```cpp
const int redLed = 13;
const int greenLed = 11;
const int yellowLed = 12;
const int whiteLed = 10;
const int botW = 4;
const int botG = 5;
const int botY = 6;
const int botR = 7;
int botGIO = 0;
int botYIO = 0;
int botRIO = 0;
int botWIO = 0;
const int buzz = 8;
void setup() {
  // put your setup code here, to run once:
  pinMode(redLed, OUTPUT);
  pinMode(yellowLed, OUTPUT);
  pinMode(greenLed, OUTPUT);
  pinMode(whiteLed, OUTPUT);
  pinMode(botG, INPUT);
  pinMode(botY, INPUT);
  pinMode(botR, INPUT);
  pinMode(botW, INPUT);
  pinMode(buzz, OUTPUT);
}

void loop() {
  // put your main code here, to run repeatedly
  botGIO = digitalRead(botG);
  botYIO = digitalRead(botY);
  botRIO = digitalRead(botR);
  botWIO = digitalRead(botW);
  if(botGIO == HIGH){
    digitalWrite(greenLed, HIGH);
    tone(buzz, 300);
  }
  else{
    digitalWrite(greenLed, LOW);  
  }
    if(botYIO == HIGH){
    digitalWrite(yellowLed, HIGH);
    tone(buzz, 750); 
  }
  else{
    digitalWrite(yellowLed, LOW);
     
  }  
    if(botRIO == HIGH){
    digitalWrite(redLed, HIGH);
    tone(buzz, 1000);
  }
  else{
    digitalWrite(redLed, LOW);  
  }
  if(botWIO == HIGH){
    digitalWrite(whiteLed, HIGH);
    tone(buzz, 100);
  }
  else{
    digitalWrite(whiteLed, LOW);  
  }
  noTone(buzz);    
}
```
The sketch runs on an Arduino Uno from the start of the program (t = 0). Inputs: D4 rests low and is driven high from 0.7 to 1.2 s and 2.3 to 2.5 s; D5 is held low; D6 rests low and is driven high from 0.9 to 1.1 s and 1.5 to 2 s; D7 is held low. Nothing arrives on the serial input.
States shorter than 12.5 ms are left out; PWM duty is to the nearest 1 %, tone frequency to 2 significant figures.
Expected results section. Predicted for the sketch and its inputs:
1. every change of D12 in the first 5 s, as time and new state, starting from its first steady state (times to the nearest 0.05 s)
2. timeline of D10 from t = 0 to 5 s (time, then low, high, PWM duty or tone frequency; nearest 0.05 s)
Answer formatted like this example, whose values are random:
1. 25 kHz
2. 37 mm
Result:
1. 0 s low; 0.9 s high; 1.1 s low; 1.5 s high; 2 s low
2. 0 s low; 0.7 s high; 1.2 s low; 2.3 s high; 2.5 s low
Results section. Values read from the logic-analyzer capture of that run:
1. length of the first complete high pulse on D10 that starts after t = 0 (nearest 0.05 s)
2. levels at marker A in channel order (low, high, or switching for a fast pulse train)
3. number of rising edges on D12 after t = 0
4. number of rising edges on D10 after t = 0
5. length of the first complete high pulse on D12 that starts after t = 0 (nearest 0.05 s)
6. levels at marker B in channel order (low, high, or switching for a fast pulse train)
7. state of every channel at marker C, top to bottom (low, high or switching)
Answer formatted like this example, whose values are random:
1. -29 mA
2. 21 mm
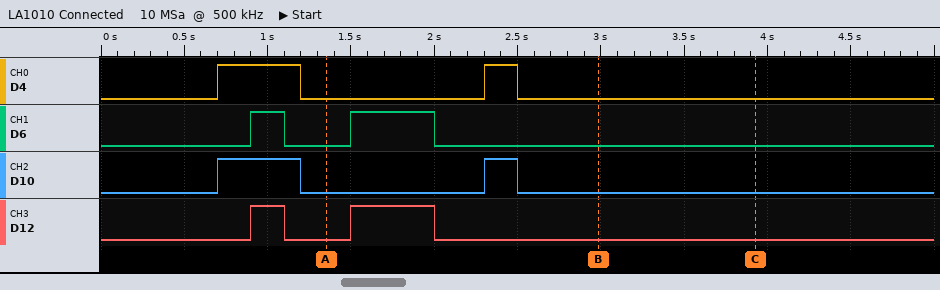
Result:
1. 0.50 s
2. D4 low, D6 low, D10 low, D12 low
3. 2
4. 2
5. 0.20 s
6. D4 low, D6 low, D10 low, D12 low
7. D4 low, D6 low, D10 low, D12 low
